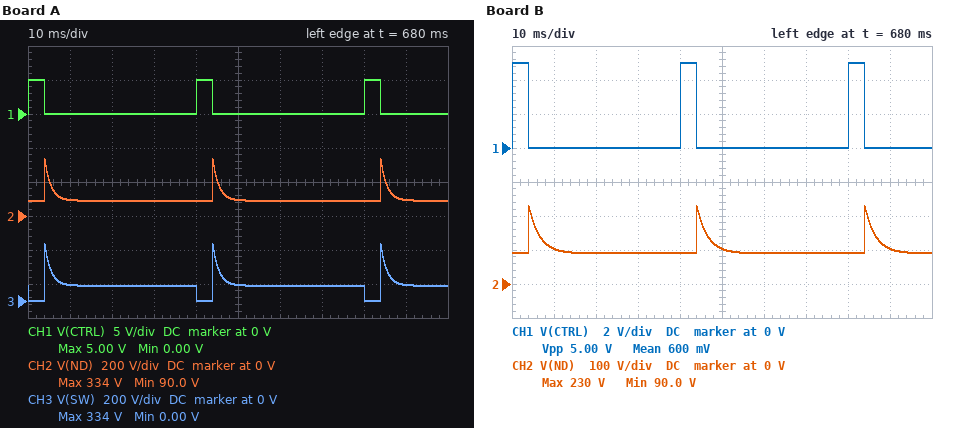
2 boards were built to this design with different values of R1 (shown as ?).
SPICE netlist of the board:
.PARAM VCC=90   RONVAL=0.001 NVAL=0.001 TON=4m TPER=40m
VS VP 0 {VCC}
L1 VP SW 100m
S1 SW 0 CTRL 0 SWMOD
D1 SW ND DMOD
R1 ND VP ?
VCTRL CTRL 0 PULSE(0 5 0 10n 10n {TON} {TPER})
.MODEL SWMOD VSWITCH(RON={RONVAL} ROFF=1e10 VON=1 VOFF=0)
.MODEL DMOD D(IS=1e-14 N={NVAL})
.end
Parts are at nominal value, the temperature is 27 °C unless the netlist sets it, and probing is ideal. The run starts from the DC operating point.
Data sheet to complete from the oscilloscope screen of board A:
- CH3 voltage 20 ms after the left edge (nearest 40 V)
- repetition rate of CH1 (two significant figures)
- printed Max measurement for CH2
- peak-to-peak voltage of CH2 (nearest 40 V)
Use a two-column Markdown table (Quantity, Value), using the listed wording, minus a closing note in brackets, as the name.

| Quantity | Value |
|---|---|
| CH3 voltage 20 ms after the left edge | 80 V |
| repetition rate of CH1 | 25 Hz |
| printed Max measurement for CH2 | 334 V |
| peak-to-peak voltage of CH2 | 240 V |
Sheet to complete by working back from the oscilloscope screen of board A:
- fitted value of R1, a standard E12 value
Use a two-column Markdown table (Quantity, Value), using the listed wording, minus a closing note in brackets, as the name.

| Quantity | Value |
|---|---|
| fitted value of R1, a standard E12 value | 68 Ω |
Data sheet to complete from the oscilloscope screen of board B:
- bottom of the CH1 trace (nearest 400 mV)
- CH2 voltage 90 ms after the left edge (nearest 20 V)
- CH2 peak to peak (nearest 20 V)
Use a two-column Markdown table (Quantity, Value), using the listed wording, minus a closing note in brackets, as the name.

| Quantity | Value |
|---|---|
| bottom of the CH1 trace | 0 V |
| CH2 voltage 90 ms after the left edge | 100 V |
| CH2 peak to peak | 140 V |
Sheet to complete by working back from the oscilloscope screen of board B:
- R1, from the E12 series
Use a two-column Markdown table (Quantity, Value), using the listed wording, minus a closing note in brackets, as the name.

| Quantity | Value |
|---|---|
| R1, from the E12 series | 39 Ω |
